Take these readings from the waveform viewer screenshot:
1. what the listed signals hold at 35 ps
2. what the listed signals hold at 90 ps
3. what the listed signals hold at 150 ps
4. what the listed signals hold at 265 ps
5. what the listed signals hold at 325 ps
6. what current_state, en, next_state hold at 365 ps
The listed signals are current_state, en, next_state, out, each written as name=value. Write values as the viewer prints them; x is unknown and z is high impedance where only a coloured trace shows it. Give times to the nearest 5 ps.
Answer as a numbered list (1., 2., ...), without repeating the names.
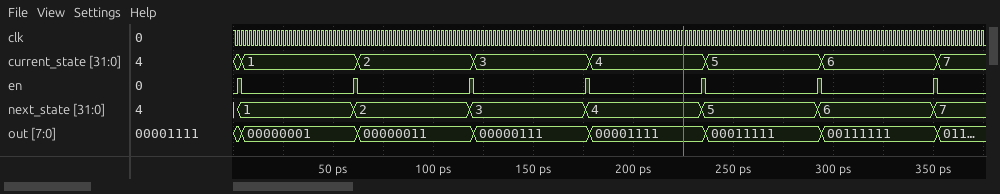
1. current_state=1, en=0, next_state=1, out=00000001
2. current_state=2, en=0, next_state=2, out=00000011
3. current_state=3, en=0, next_state=3, out=00000111
4. current_state=5, en=0, next_state=5, out=00011111
5. current_state=6, en=0, next_state=6, out=00111111
6. current_state=7, en=0, next_state=7
